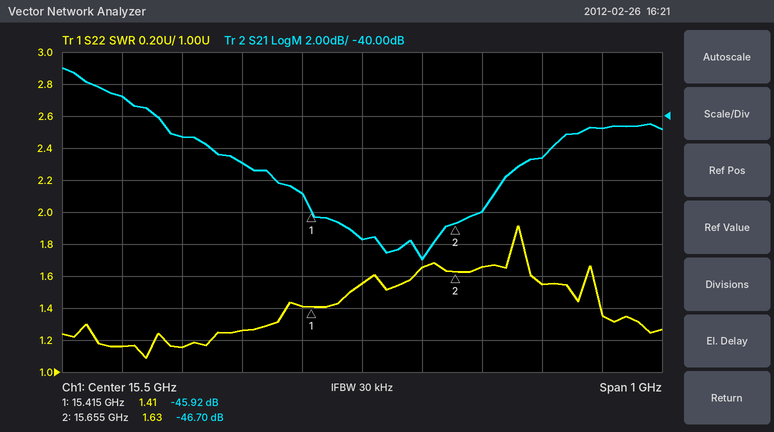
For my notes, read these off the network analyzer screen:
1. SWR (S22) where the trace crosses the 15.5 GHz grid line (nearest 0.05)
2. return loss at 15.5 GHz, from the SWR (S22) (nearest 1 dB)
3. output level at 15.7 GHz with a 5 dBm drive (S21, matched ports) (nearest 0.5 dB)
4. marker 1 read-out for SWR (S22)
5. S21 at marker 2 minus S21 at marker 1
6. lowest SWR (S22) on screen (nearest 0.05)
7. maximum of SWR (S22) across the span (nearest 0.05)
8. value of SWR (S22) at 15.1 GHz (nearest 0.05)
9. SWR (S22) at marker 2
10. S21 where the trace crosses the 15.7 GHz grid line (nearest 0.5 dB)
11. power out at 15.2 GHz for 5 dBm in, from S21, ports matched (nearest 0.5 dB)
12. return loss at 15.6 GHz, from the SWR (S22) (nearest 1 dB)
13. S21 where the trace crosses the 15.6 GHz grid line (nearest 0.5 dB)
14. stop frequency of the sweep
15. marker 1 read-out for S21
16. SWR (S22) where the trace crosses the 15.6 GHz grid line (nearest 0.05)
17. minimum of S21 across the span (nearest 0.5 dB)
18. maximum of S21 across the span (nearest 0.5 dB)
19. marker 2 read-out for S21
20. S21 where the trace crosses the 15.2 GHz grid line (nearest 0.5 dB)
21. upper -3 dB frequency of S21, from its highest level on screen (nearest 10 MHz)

1.55
13 dB
-41.0 dBm
1.41
-0.78 dB
1.10
1.90
1.15
1.63
-46.0 dB
-36.5 dBm
12 dB
-49.0 dB
16 GHz
-45.92 dB
1.65
-49.0 dB
-37.0 dB
-46.70 dB
-41.5 dB
15.16 GHz
